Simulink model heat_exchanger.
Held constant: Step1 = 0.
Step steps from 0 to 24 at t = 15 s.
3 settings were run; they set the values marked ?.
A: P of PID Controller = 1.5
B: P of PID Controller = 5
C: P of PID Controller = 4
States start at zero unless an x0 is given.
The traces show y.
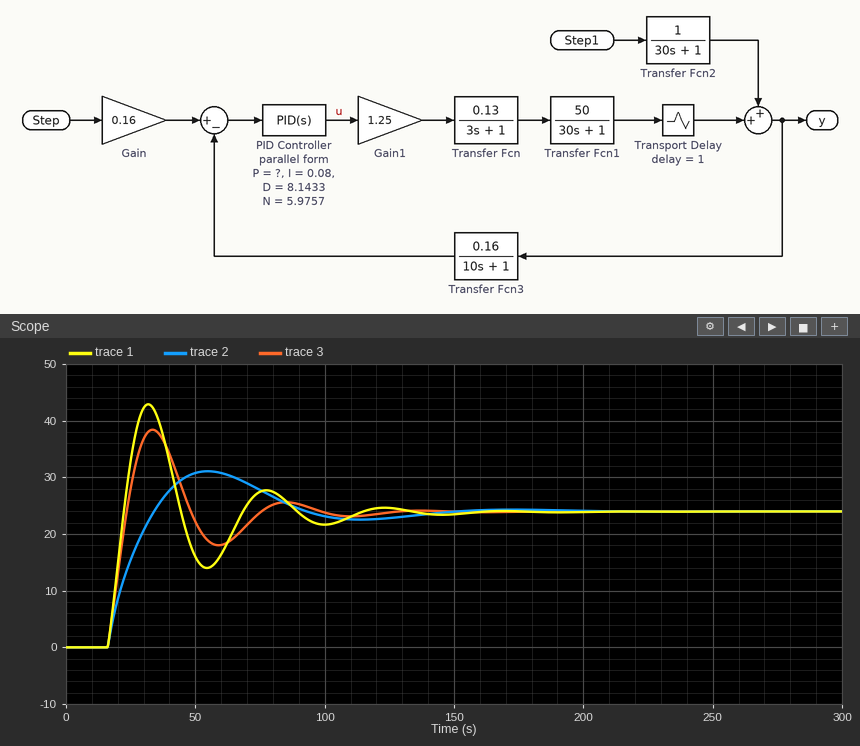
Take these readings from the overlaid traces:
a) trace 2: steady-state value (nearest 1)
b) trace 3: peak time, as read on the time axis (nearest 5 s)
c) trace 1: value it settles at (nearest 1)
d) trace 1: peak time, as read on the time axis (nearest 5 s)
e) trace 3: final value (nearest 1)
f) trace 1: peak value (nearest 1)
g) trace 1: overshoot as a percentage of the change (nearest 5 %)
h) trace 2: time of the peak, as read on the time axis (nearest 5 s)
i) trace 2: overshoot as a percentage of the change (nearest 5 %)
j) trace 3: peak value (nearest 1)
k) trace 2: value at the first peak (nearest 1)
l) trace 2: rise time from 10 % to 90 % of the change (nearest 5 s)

24
35 s
24
30 s
24
43
80 %
55 s
30 %
38
31
15 s
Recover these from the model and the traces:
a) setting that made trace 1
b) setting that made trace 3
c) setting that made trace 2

B
C
A
